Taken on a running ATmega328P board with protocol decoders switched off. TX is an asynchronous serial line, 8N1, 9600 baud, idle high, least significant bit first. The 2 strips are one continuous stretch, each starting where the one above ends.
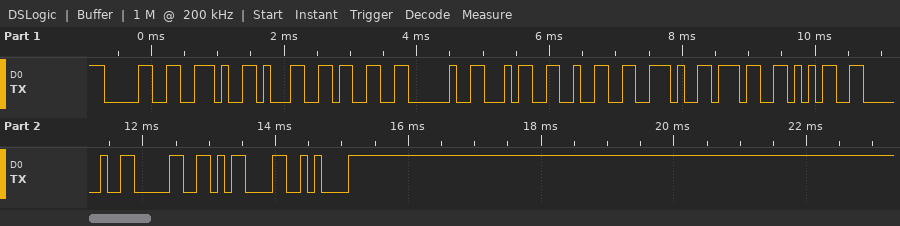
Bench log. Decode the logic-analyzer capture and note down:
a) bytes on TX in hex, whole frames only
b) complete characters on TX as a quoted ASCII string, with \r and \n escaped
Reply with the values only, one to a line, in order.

0x30 0x2E 0x31 0x33 0x20 0x34 0x32 0x2E 0x37 0x35 0x20 0x30 0x0D 0x0A
"0.13 42.75 0\r\n"
